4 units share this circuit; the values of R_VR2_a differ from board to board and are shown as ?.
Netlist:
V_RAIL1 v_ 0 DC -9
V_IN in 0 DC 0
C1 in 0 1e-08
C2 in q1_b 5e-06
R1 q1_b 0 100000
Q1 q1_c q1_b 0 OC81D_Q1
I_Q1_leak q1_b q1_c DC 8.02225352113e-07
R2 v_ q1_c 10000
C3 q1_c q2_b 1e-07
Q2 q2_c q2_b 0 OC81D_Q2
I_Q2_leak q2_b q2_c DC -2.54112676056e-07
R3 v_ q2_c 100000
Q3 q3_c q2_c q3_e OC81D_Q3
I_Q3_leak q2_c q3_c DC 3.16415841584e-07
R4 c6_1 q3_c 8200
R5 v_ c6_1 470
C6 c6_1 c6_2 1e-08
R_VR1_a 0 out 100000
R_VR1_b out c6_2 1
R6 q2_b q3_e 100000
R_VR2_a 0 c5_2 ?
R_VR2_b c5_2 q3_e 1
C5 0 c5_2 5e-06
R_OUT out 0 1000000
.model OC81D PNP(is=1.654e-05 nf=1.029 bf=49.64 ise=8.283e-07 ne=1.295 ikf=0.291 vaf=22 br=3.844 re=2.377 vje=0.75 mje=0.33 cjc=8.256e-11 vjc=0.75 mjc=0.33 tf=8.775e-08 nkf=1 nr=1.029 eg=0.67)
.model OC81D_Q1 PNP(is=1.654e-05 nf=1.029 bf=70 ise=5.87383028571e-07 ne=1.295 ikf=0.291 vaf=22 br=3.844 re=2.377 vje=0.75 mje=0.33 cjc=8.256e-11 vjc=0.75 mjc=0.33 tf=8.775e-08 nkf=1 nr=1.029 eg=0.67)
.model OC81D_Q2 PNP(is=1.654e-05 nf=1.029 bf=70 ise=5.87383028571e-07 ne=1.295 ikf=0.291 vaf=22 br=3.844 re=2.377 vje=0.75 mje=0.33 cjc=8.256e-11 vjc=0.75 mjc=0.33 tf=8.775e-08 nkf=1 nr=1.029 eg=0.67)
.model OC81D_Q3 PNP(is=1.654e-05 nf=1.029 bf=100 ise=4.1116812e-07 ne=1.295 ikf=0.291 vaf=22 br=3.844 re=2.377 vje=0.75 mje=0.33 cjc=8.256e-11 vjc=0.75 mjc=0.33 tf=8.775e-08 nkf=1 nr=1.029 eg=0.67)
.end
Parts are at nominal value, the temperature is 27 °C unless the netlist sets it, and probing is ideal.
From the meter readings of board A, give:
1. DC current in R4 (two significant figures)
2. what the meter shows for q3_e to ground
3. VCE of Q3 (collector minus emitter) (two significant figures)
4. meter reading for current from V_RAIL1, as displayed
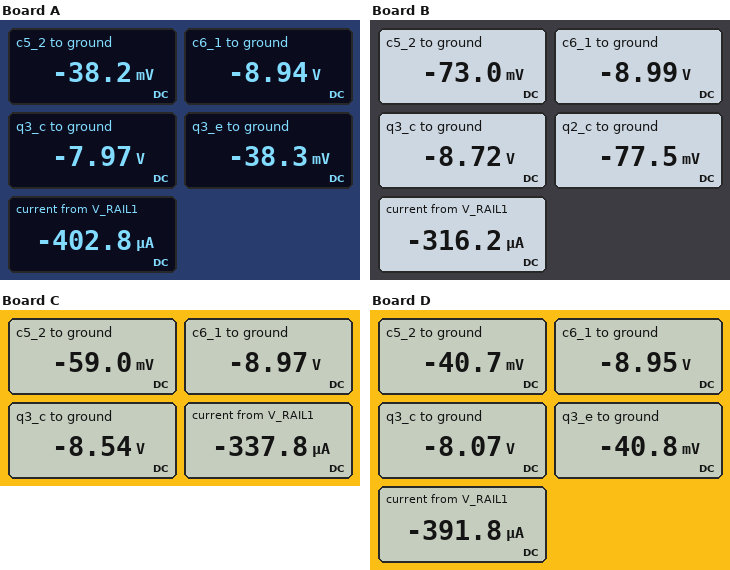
120 µA
-38.3 mV
-7.9 V
-402.8 µA
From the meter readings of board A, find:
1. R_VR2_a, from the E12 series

330 Ω
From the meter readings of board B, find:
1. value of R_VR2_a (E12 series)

2.7 kΩ
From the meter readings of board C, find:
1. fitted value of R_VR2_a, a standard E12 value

1.2 kΩ
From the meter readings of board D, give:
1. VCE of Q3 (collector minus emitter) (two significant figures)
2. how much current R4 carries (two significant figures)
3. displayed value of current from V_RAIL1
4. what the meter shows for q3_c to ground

-8.0 V
110 µA
-391.8 µA
-8.07 V
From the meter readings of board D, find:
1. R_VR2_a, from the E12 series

390 Ω
